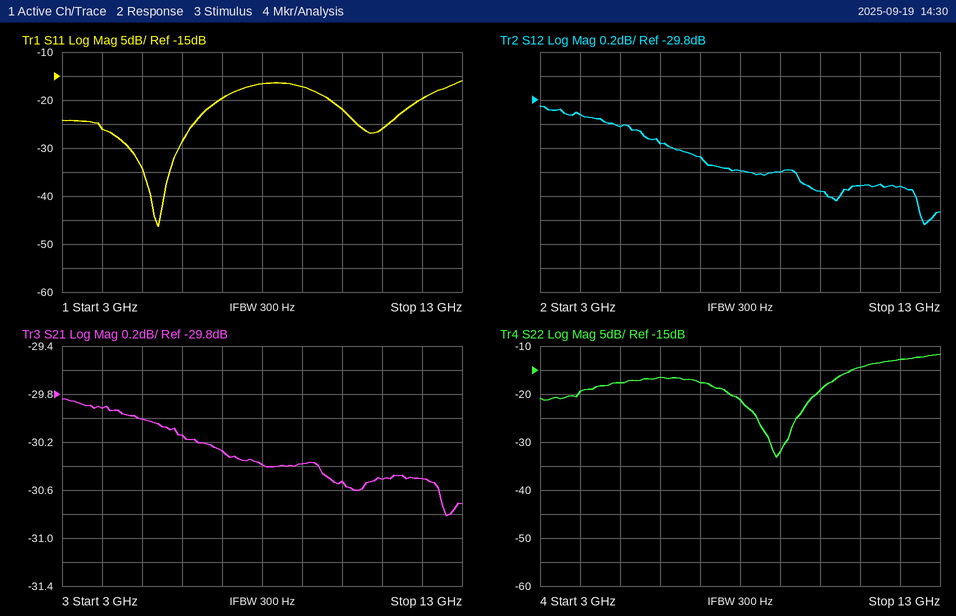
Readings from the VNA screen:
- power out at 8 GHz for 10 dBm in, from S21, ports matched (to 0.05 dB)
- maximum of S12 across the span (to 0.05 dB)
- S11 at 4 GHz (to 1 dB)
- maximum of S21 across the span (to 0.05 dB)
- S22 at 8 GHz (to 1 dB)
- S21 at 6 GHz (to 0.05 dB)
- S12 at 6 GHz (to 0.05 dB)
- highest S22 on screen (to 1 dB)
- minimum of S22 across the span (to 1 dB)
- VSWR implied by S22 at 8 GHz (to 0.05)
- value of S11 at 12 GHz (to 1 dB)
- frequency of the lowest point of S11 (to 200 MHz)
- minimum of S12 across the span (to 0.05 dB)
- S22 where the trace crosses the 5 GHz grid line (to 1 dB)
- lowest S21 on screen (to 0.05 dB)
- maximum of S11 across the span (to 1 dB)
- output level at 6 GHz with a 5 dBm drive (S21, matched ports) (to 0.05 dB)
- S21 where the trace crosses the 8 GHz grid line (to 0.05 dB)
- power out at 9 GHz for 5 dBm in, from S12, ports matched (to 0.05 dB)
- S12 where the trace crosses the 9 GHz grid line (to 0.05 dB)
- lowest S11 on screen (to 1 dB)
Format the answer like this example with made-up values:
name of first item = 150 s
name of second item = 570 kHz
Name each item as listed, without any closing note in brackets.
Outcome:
power out at 8 GHz for 10 dBm in, from S21, ports matched = -20.40 dBm
maximum of S12 across the span = -29.85 dB
S11 at 4 GHz = -26 dB
maximum of S21 across the span = -29.85 dB
S22 at 8 GHz = -21 dB
S21 at 6 GHz = -30.15 dB
S12 at 6 GHz = -30.15 dB
highest S22 on screen = -12 dB
minimum of S22 across the span = -33 dB
VSWR implied by S22 at 8 GHz = 1.20
value of S11 at 12 GHz = -20 dB
frequency of the lowest point of S11 = 5.4 GHz
minimum of S12 across the span = -30.85 dB
S22 where the trace crosses the 5 GHz grid line = -18 dB
lowest S21 on screen = -30.80 dB
maximum of S11 across the span = -16 dB
output level at 6 GHz with a 5 dBm drive (S21, matched ports) = -25.15 dBm
S21 where the trace crosses the 8 GHz grid line = -30.40 dB
power out at 9 GHz for 5 dBm in, from S12, ports matched = -25.40 dBm
S12 where the trace crosses the 9 GHz grid line = -30.40 dB
lowest S11 on screen = -46 dB
